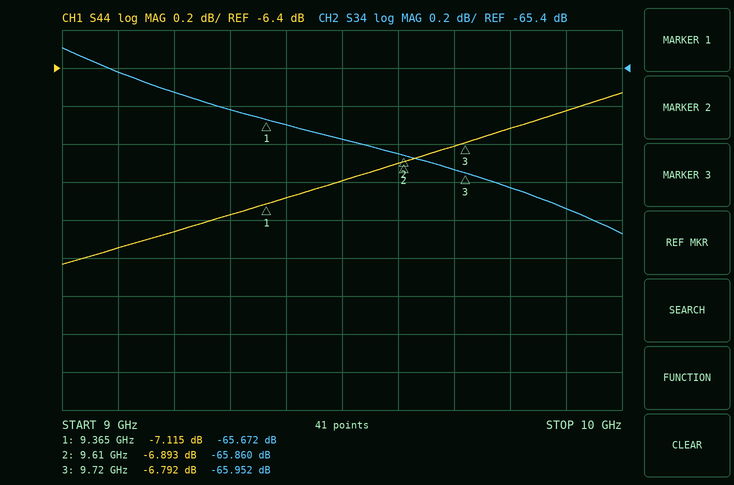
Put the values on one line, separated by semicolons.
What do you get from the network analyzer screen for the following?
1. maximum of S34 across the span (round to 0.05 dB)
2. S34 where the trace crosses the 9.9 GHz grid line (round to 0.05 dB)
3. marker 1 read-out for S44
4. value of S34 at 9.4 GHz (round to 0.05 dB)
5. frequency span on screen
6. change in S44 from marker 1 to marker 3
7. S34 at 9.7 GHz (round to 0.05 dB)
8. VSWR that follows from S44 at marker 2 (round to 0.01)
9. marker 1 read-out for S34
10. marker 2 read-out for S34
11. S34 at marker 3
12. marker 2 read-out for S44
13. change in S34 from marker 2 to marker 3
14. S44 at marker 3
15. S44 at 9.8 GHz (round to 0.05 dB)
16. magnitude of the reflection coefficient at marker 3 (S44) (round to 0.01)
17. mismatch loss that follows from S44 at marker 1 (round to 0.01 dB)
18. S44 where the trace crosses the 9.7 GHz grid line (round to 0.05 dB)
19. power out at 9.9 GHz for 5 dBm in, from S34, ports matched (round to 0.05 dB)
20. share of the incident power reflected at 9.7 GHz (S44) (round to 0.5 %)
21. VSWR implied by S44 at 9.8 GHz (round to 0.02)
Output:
-65.30 dB; -66.15 dB; -7.115 dB; -65.70 dB; 1 GHz; 0.323 dB; -65.95 dB; 2.65; -65.672 dB; -65.860 dB; -65.952 dB; -6.893 dB; -0.092 dB; -6.792 dB; -6.70 dB; 0.46; 0.94 dB; -6.80 dB; -61.15 dBm; 21.0 %; 2.72
